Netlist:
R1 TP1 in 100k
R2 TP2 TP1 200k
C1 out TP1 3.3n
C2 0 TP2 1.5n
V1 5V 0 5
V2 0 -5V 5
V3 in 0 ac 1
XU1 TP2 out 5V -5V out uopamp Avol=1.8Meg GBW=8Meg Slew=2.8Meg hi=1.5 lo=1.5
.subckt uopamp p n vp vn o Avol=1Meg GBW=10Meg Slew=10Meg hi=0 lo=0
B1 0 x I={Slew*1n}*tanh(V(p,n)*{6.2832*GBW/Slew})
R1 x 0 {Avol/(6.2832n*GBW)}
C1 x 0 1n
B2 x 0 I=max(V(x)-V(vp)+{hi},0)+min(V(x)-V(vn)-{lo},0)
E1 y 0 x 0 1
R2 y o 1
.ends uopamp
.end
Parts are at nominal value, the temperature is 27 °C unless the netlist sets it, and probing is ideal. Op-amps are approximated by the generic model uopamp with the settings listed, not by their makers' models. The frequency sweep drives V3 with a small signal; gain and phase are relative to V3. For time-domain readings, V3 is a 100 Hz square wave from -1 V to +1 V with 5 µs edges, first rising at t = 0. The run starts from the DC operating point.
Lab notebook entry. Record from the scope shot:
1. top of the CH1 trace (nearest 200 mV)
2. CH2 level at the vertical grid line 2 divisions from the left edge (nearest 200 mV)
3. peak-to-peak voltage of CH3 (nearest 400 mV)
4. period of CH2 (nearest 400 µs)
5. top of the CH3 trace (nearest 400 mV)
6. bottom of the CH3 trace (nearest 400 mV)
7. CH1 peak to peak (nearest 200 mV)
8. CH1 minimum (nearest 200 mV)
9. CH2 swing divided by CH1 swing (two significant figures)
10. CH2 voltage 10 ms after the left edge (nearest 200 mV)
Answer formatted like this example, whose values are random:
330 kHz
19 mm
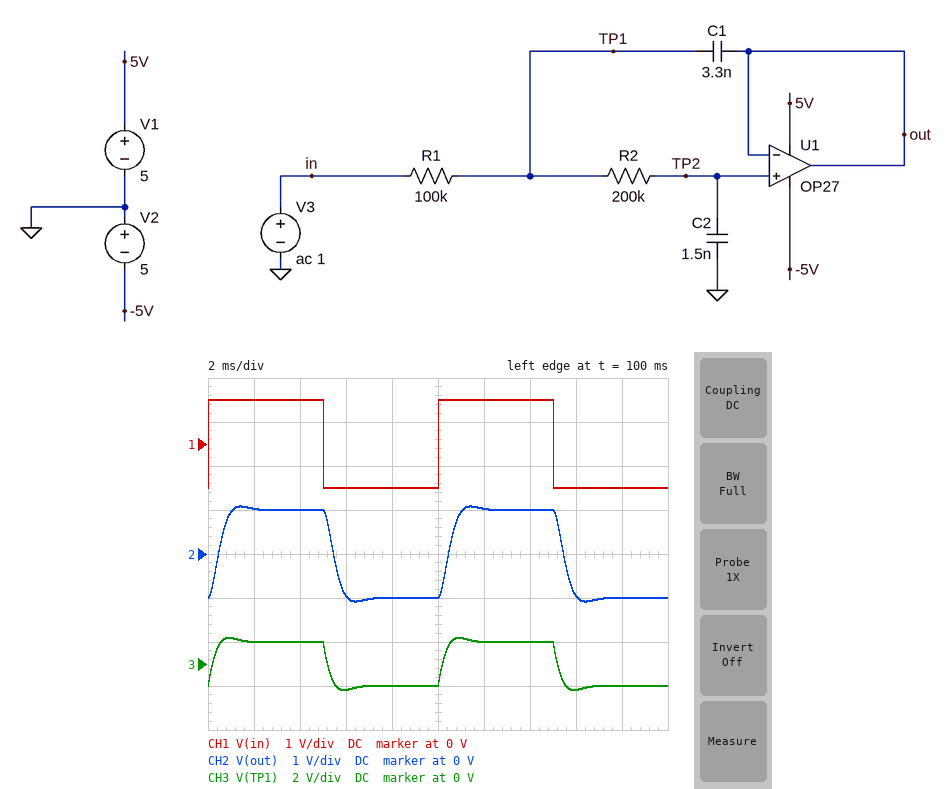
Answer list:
1.0 V
1.0 V
2.4 V
10.0 ms
1.2 V
-1.2 V
2.0 V
-1.0 V
1.1
-1.0 V
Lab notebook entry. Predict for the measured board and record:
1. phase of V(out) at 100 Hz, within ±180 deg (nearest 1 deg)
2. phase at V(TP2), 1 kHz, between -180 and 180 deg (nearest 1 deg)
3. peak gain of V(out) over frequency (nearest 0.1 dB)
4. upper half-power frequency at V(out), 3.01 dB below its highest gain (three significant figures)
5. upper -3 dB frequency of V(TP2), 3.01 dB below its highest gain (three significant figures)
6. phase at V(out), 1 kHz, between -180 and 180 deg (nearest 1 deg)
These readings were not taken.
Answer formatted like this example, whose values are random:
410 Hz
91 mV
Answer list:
-16 deg
-136 deg
0 dB
500 Hz
500 Hz
-136 deg
